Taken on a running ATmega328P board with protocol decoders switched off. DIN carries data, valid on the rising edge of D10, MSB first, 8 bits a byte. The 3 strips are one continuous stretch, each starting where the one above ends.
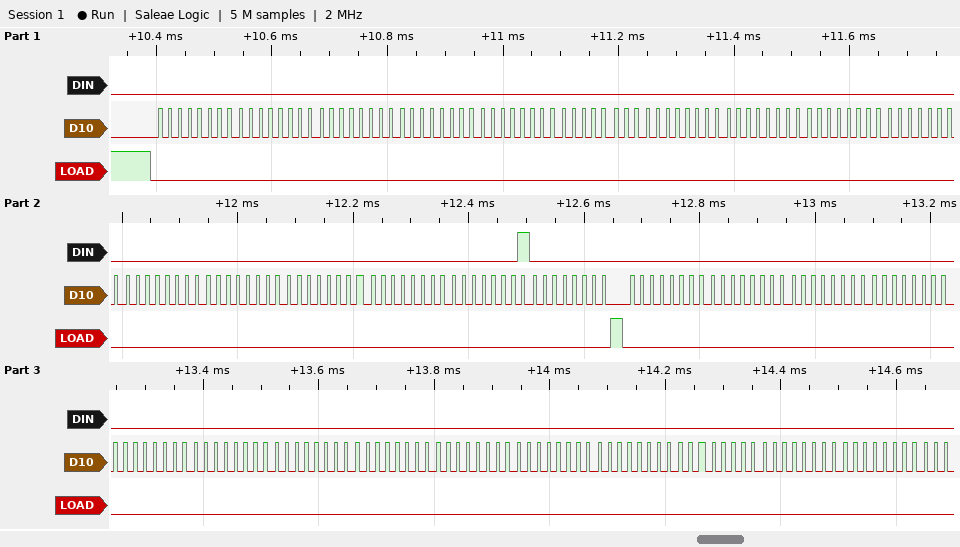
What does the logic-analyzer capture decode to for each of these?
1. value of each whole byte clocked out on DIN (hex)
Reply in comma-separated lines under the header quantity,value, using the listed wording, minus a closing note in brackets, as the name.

quantity,value
value of each whole byte clocked out on DIN,0x00 0x00 0x00 0x00 0x00 0x00 0x00 0x00 0x00 0x00 0x00 0x00 0x00 0x00 0x01 0x00 0x00 0x00 0x00 0x00 0x00 0x00 0x00 0x00 0x00 0x00 0x00 0x00 0x00 0x00
